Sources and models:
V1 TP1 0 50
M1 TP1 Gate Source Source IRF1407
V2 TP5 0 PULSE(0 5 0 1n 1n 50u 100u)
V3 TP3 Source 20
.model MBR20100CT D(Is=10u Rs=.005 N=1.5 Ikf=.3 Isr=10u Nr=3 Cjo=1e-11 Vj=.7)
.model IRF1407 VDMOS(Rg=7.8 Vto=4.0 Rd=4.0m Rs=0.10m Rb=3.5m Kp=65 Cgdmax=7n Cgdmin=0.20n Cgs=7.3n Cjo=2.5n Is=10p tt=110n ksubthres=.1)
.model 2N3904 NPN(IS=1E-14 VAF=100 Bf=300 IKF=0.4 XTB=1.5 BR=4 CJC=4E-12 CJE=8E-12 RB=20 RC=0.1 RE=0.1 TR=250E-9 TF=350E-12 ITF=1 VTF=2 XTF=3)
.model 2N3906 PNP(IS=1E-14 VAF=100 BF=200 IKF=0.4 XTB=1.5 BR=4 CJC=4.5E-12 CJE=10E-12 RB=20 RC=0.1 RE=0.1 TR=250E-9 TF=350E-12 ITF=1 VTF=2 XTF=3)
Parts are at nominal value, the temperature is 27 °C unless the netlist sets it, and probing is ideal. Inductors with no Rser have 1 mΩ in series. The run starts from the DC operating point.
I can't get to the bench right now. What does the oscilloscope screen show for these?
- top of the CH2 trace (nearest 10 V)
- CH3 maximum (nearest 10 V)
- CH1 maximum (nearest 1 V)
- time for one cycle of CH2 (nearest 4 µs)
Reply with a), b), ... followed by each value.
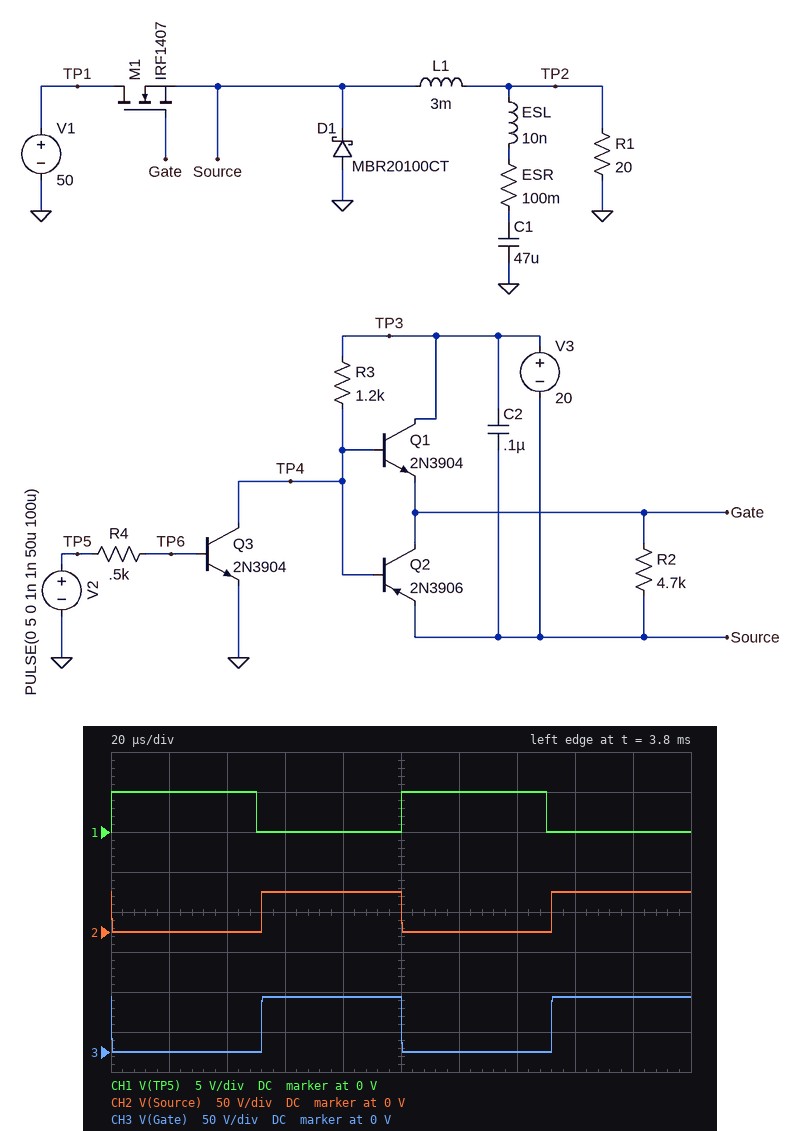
a) 50 V
b) 70 V
c) 5 V
d) 100 µs
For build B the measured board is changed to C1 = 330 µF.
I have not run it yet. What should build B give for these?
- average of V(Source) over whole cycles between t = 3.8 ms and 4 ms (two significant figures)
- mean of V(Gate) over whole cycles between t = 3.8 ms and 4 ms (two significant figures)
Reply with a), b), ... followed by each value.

a) 25 V
b) 34 V
